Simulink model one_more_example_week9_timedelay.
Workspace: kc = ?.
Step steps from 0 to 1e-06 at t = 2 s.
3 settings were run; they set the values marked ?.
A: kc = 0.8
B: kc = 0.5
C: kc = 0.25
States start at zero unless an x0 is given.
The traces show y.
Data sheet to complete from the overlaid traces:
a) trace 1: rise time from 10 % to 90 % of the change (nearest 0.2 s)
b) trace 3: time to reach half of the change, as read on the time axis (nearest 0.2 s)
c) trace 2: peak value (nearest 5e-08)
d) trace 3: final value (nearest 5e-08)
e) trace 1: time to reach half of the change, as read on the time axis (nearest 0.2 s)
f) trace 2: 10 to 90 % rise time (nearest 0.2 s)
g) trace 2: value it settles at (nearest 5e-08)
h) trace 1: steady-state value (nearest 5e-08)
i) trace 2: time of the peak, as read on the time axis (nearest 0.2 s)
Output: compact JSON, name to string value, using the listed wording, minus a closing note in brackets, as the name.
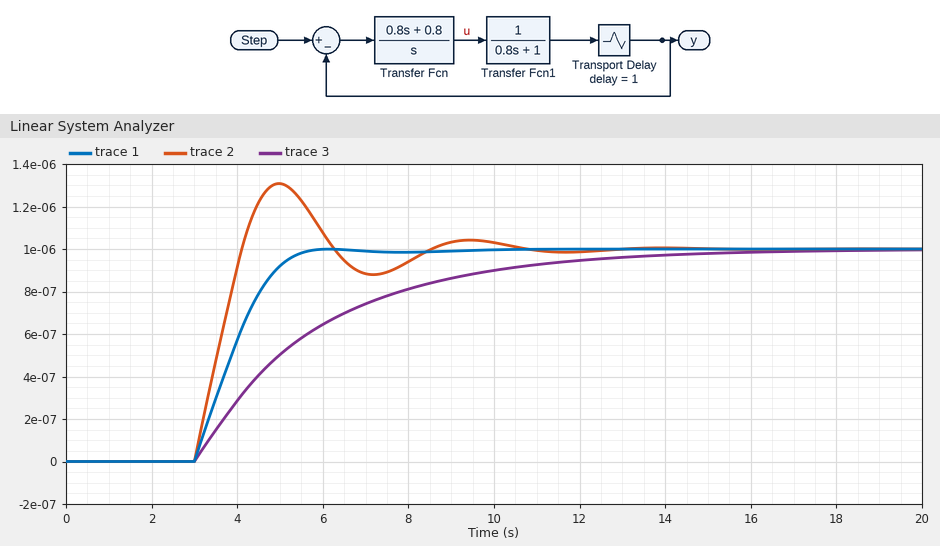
{"trace 1: rise time from 10 % to 90 % of the change": "1.8 s", "trace 3: time to reach half of the change, as read on the time axis": "5.0 s", "trace 2: peak value": "0.00000130", "trace 3: final value": "0.00000100", "trace 1: time to reach half of the change, as read on the time axis": "3.8 s", "trace 2: 10 to 90 % rise time": "0.8 s", "trace 2: value it settles at": "0.00000100", "trace 1: steady-state value": "0.00000100", "trace 2: time of the peak, as read on the time axis": "5.0 s"}
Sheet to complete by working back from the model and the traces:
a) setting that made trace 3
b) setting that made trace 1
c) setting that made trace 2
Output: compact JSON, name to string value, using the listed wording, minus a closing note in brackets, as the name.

{"setting that made trace 3": "C", "setting that made trace 1": "B", "setting that made trace 2": "A"}
